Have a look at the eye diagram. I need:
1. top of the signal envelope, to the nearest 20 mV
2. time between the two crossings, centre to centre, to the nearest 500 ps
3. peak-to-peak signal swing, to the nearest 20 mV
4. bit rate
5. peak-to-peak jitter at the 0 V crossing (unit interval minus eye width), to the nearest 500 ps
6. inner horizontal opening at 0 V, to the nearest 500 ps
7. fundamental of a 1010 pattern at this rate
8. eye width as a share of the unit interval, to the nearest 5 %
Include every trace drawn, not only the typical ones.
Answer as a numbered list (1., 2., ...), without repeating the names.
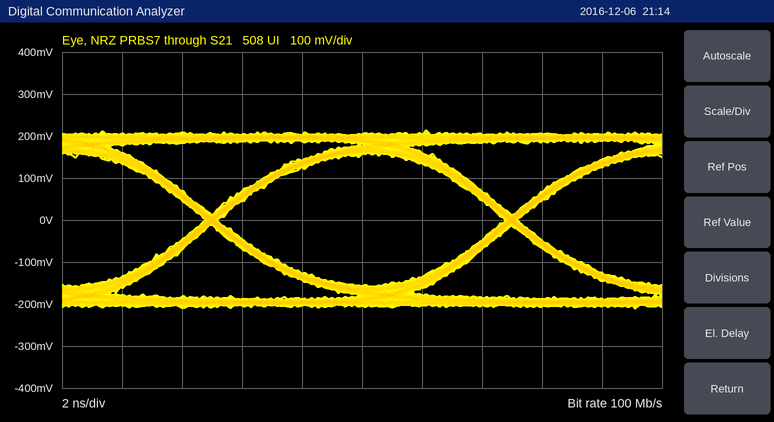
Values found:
1. 220 mV
2. 10.0 ns
3. 420 mV
4. 100 Mb/s
5. 500 ps
6. 9.5 ns
7. 50 MHz
8. 95 %
